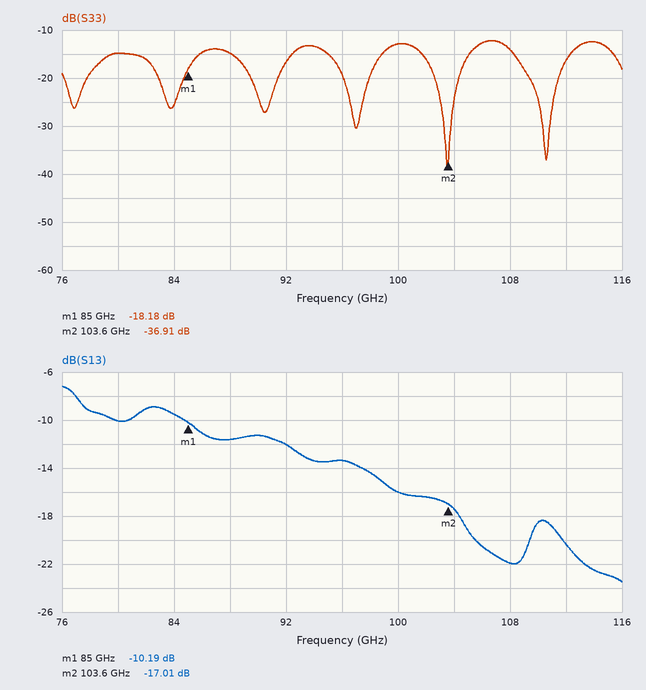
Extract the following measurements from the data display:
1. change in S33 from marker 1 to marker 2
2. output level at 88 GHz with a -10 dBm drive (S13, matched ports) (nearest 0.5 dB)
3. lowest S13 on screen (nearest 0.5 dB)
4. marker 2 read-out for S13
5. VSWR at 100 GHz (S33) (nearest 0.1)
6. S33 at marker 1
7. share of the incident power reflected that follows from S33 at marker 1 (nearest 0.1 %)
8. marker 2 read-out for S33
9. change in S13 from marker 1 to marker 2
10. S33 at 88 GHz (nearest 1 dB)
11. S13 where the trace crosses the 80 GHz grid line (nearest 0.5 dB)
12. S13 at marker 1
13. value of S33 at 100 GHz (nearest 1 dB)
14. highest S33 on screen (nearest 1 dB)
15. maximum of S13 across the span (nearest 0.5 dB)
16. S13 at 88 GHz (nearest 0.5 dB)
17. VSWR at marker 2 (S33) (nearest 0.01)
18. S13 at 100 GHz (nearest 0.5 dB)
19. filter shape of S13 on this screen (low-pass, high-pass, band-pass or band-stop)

-18.73 dB
-21.5 dBm
-23.5 dB
-17.01 dB
1.6
-18.18 dB
1.5 %
-36.91 dB
-6.82 dB
-15 dB
-10.0 dB
-10.19 dB
-13 dB
-12 dB
-7.0 dB
-11.5 dB
1.03
-16.0 dB
low-pass
